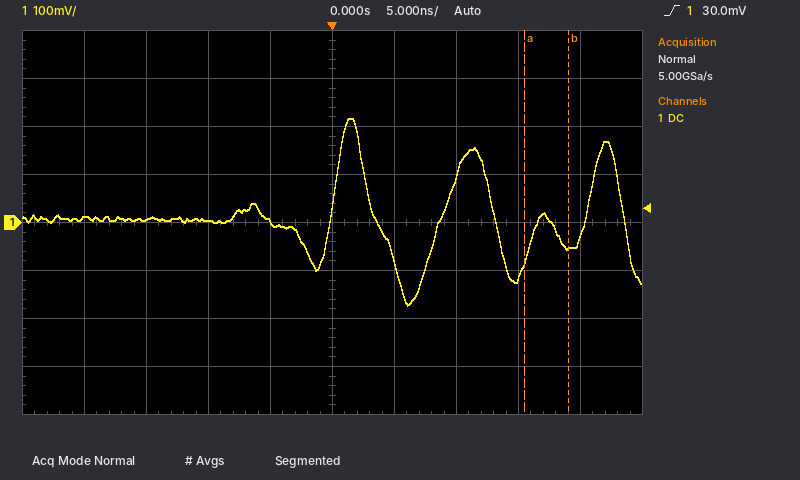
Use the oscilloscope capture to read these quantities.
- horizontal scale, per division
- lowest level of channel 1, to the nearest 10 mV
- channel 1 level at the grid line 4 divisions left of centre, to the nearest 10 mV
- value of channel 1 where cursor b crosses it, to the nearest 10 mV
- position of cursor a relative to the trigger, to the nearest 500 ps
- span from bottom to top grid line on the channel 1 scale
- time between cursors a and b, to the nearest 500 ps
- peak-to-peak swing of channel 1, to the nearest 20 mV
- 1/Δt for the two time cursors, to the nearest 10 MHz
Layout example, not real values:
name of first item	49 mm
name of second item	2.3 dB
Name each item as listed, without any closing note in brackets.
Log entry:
horizontal scale, per division	5 ns
lowest level of channel 1, to the nearest 10 mV	-170 mV
channel 1 level at the grid line 4 divisions left of centre, to the nearest 10 mV	10 mV
value of channel 1 where cursor b crosses it, to the nearest 10 mV	-50 mV
position of cursor a relative to the trigger, to the nearest 500 ps	+15.5 ns
span from bottom to top grid line on the channel 1 scale	800 mV
time between cursors a and b, to the nearest 500 ps	3.5 ns
peak-to-peak swing of channel 1, to the nearest 20 mV	380 mV
1/Δt for the two time cursors, to the nearest 10 MHz	290 MHz
